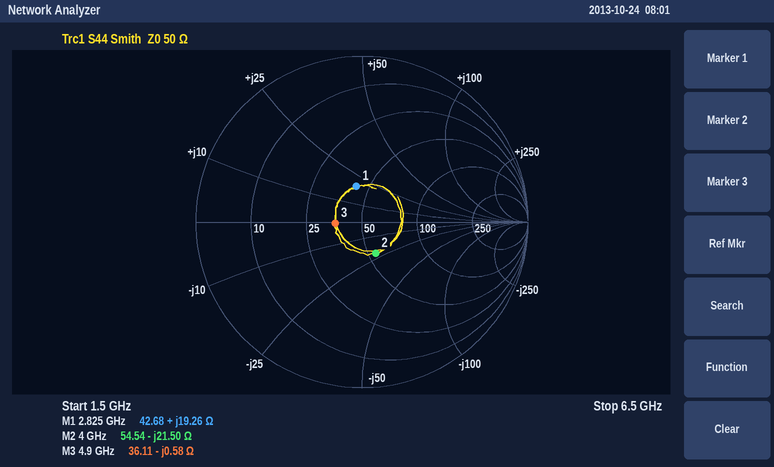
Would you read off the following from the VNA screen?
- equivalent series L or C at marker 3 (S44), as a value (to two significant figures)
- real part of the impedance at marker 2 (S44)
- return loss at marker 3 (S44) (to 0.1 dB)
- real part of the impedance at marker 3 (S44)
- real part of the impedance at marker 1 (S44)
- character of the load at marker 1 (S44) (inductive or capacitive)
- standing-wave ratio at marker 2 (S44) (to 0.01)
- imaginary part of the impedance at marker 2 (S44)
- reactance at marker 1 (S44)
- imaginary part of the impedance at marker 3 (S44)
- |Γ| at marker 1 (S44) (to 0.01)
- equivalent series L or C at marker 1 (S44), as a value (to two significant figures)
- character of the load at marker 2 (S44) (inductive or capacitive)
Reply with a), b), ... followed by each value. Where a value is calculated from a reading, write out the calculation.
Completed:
a) C = 1/(2π × 4.9 GHz × 0.58 Ω) ≈ 56 pF
b) 54.54 Ω
c) 15.8 dB
d) 36.11 Ω
e) 42.68 Ω
f) inductive
g) 1.52
h) -21.50 Ω
i) +19.26 Ω
j) -0.58 Ω
k) 0.22
l) L = 19.26 Ω/(2π × 2.825 GHz) ≈ 1.1 nH
m) capacitive
